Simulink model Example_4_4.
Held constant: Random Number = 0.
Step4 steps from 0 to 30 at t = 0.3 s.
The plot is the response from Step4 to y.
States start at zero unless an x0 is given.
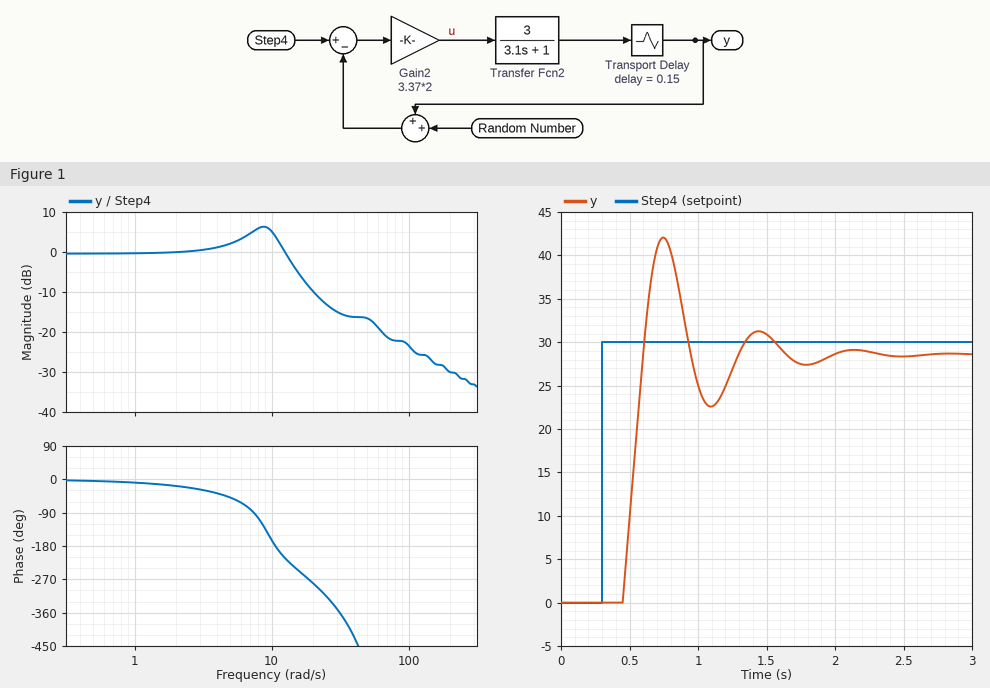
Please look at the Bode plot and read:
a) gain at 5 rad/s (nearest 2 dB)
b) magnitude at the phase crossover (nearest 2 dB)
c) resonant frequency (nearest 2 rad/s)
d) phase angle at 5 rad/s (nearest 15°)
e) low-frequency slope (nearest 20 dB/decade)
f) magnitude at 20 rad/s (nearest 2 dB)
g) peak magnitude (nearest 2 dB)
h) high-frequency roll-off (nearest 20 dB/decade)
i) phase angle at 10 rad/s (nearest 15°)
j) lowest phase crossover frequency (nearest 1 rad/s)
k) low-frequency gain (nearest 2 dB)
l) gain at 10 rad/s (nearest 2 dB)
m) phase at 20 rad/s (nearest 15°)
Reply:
2 dB
4 dB
8 rad/s
-45°
0 dB/decade
-10 dB
6 dB
-20 dB/decade
-165°
11 rad/s
0 dB
6 dB
-285°
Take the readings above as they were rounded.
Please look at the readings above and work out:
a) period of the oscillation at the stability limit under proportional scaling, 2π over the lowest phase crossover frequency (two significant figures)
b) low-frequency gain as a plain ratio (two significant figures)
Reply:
0.57 s
1.0
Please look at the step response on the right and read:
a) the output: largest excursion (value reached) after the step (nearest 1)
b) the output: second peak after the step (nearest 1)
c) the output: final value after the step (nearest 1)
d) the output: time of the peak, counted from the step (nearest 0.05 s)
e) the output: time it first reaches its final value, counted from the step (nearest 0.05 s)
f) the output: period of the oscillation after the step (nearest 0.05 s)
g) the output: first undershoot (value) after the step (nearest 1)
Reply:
42
31
29
0.45 s
0.30 s
0.70 s
23
